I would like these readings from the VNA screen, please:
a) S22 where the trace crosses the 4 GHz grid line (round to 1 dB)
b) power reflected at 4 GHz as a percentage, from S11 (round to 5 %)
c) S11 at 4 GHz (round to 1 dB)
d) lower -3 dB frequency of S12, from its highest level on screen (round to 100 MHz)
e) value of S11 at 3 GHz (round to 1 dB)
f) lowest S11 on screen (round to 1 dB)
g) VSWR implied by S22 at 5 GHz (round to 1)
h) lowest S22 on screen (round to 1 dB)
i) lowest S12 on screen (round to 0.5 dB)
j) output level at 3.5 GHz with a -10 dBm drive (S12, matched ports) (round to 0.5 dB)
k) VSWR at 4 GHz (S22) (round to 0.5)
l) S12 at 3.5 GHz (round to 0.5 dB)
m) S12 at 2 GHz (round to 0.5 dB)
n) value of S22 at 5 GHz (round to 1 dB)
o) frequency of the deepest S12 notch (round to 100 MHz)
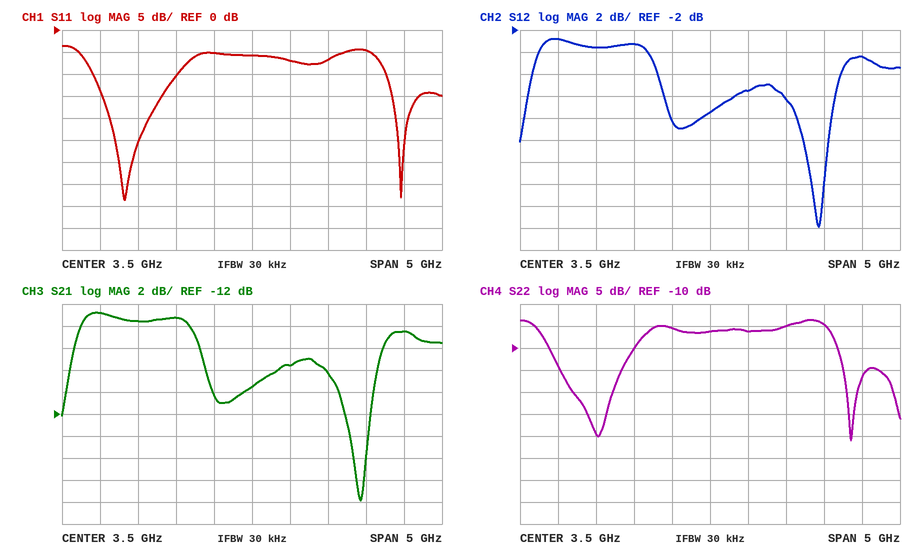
-6 dB
20 %
-7 dB
1.2 GHz
-5 dB
-39 dB
4
-31 dB
-20.0 dB
-19.5 dBm
3.0
-9.5 dB
-3.5 dB
-5 dB
4.9 GHz
